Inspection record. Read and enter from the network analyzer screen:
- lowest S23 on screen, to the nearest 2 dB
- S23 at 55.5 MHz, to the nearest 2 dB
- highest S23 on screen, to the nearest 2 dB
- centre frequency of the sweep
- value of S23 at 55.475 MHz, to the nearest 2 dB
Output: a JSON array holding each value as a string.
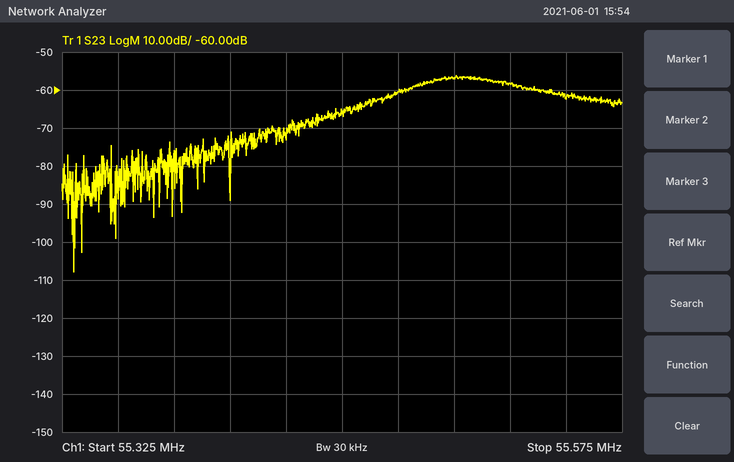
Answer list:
["-108 dB", "-56 dB", "-56 dB", "55.45 MHz", "-60 dB"]
